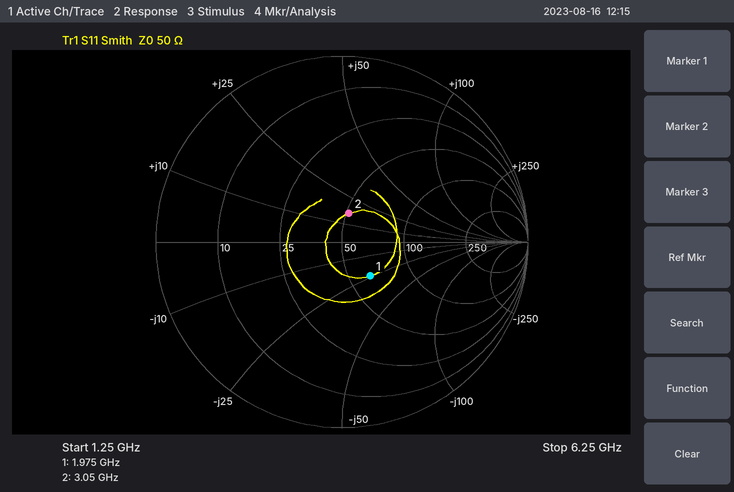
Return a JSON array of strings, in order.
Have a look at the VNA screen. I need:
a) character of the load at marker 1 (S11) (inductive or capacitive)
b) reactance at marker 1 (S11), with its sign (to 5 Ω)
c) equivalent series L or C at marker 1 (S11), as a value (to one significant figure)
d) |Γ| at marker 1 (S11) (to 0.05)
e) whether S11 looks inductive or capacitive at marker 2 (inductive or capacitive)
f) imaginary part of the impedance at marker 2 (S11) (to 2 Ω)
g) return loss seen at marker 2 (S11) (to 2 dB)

["capacitive", "-25 Ω", "3 pF", "0.25", "inductive", "+16 Ω", "16 dB"]
